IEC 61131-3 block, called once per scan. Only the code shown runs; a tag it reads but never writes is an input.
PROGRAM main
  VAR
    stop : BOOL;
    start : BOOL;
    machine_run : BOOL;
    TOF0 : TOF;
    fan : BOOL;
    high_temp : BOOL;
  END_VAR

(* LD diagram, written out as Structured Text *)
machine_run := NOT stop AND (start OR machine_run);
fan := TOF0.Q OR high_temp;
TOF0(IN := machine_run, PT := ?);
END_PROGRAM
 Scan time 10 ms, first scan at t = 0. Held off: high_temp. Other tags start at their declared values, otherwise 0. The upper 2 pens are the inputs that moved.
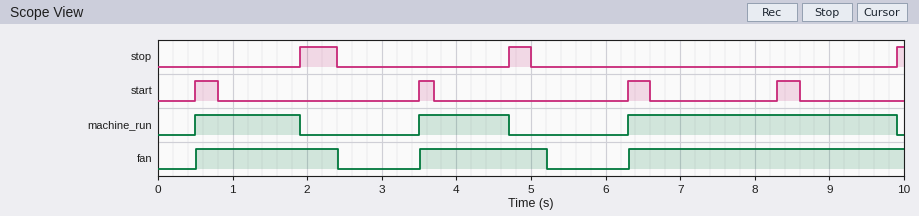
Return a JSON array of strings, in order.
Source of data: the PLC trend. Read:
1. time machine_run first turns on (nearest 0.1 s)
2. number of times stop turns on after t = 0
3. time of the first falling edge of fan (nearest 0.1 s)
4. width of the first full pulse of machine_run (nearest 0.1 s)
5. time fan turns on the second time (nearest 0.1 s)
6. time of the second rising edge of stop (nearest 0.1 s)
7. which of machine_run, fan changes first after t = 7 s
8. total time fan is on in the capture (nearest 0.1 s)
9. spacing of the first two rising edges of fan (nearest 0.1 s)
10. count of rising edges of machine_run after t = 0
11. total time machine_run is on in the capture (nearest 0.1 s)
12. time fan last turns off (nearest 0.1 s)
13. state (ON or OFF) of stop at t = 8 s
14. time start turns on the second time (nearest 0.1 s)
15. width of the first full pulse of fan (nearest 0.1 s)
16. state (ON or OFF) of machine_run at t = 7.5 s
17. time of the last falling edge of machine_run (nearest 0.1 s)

["0.5 s", "3", "2.4 s", "1.4 s", "3.5 s", "4.7 s", "machine_run", "7.3 s", "3.0 s", "3", "6.2 s", "5.2 s", "OFF", "3.5 s", "1.9 s", "ON", "9.9 s"]
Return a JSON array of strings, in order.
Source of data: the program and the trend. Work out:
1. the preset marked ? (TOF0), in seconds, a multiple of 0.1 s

["0.5 s"]
